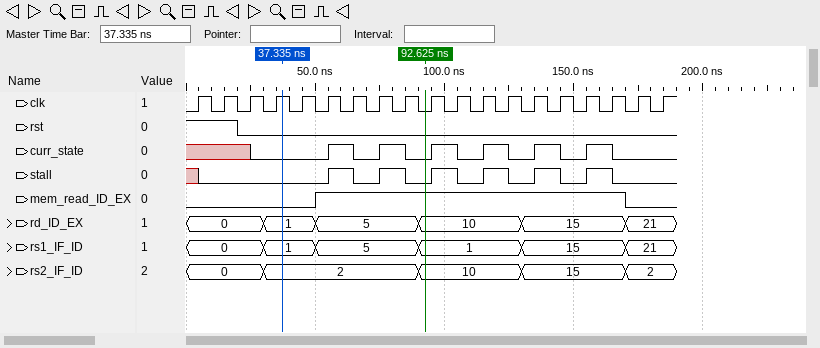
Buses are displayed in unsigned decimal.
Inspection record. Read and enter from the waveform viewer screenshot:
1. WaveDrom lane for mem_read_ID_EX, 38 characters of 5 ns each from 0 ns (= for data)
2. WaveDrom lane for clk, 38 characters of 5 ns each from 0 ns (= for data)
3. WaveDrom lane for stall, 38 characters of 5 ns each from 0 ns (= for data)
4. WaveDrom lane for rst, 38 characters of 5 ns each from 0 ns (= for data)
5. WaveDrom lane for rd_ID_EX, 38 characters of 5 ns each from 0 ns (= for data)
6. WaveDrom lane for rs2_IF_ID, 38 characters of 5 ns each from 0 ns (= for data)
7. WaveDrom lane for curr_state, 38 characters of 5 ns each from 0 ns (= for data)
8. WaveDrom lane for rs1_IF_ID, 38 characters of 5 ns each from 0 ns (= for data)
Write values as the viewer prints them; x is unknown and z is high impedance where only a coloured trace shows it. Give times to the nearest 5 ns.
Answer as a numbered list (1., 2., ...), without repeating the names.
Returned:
1. {name: 'mem_read_ID_EX', wave: '0.........1.......................0...'}
2. {name: 'clk', wave: '01010101010101010101010101010101010101'}
3. {name: 'stall', wave: 'x0.........1.0.1.0.1.0.1.0.1.0.1.0....'}
4. {name: 'rst', wave: '1...0.................................'}
5. {name: 'rd_ID_EX', wave: '=.....=...=.......=.......=.......=...', data: '0 1 5 10 15 21'}
6. {name: 'rs2_IF_ID', wave: '=.....=...........=.......=.......=...', data: '0 2 10 15 2'}
7. {name: 'curr_state', wave: 'x....0.....1.0.1.0.1.0.1.0.1.0.1.0....'}
8. {name: 'rs1_IF_ID', wave: '=.....=...=.......=.......=.......=...', data: '0 1 5 1 15 21'}
